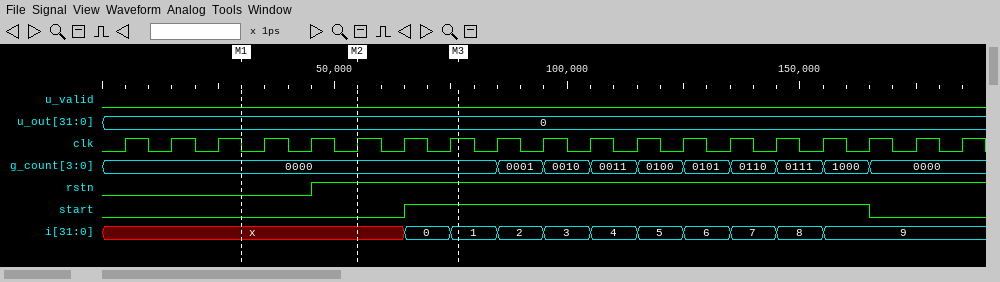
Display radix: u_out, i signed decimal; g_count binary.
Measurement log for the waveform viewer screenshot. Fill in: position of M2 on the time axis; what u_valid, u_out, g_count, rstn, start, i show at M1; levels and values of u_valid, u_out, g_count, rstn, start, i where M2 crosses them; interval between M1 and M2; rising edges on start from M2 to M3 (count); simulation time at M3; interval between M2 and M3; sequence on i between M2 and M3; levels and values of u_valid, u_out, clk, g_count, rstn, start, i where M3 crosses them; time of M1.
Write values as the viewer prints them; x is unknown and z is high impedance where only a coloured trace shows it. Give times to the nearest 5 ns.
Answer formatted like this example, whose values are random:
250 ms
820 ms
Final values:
55 ns
u_valid=0, u_out=0, g_count=0000, rstn=0, start=0, i=x
u_valid=0, u_out=0, g_count=0000, rstn=1, start=0, i=x
25 ns
1
75 ns
20 ns
x, 0, 1
u_valid=0, u_out=0, clk=1, g_count=0000, rstn=1, start=1, i=1
30 ns
